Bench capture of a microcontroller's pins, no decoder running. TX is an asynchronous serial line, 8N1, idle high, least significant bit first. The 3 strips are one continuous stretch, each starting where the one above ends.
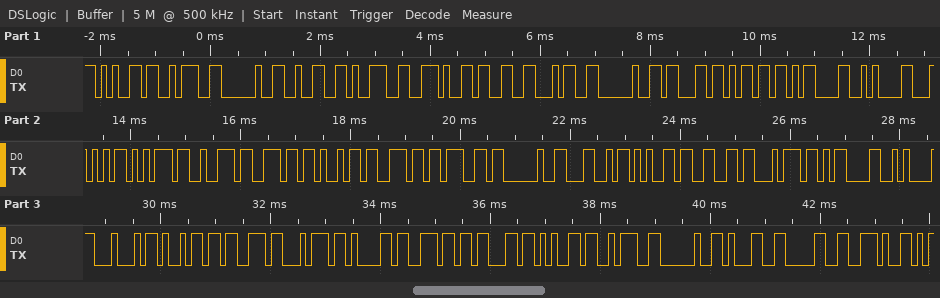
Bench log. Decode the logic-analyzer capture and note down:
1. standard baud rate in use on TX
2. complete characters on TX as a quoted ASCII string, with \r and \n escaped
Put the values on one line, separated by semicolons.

9600 baud; "e: 29.34 cm\r\nTurning Left\r\nDistance: 10."
